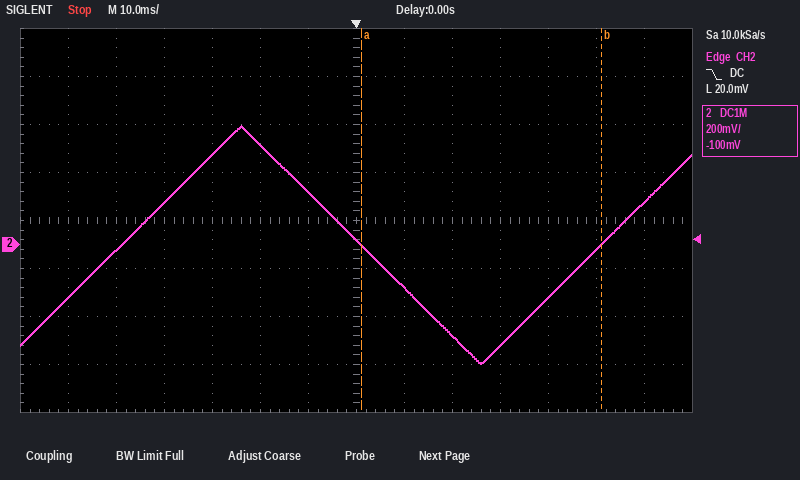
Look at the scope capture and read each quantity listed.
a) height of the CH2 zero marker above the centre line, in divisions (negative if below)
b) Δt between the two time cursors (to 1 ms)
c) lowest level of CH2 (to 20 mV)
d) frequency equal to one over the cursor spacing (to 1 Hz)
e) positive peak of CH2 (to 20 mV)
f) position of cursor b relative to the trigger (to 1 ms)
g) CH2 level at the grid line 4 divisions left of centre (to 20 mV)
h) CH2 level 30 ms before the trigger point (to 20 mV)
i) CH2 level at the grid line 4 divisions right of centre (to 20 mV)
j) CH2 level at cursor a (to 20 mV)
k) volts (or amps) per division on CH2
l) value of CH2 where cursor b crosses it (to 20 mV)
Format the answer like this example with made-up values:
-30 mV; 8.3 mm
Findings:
-0.5 div; 50 ms; -500 mV; 20 Hz; 500 mV; +51 ms; 180 mV; 380 mV; -220 mV; 0 mV; 200 mV; 0 mV
